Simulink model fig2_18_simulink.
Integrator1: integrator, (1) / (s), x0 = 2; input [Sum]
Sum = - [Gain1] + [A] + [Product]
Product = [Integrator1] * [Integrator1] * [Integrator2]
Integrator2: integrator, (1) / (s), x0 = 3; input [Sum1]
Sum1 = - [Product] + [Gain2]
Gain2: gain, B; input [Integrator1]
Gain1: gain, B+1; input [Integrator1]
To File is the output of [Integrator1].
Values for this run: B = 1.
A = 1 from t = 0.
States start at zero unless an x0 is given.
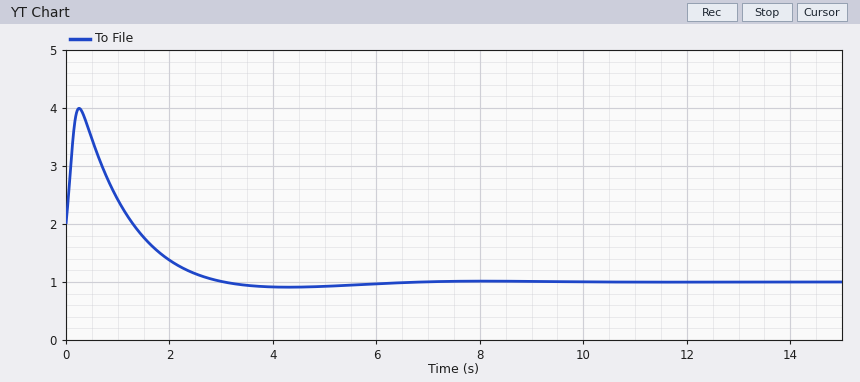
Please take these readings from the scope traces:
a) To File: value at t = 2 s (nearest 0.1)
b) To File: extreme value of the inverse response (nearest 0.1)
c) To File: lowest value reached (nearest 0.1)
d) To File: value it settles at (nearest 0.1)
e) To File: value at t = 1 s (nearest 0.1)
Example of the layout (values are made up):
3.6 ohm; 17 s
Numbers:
1.4; 4.0; 0.9; 1.0; 2.4
